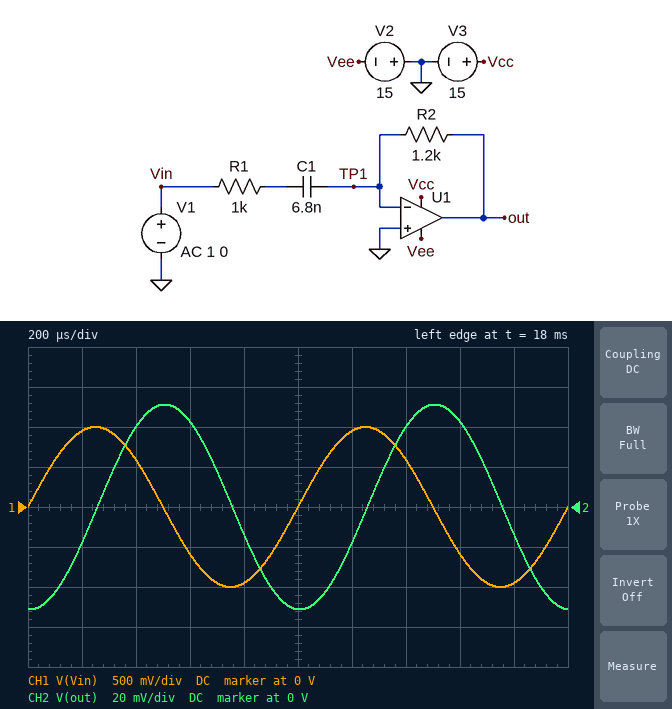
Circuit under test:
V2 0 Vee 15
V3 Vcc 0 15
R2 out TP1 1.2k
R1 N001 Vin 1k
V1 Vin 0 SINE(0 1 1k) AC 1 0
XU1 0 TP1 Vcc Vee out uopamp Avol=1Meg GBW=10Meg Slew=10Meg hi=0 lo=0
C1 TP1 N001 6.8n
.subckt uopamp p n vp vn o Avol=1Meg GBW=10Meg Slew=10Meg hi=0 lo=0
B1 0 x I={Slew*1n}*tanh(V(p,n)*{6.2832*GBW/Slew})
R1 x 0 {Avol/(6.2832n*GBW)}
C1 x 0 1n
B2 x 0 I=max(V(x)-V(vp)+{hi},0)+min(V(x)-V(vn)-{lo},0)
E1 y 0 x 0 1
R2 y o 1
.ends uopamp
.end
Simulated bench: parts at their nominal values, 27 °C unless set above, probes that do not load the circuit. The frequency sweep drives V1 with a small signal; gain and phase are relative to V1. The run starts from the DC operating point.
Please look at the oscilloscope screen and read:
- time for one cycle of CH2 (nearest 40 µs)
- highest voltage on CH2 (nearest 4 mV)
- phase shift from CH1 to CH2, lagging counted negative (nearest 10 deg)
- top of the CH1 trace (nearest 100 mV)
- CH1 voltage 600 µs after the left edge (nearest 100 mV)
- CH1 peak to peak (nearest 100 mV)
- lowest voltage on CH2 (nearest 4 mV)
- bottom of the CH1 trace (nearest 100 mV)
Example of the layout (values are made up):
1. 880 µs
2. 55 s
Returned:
1. 1.00 ms
2. 52 mV
3. -90 deg
4. 1.0 V
5. -600 mV
6. 2.0 V
7. -52 mV
8. -1.0 V
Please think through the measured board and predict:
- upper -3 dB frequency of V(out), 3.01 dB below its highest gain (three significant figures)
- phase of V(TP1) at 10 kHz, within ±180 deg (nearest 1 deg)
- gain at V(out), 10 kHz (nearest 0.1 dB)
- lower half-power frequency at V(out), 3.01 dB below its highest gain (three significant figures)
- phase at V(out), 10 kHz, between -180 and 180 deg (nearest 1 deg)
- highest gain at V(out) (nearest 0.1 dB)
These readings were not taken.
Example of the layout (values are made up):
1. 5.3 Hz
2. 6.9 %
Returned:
1. 4.58 MHz
2. 157 deg
3. -6.5 dB
4. 23.2 kHz
5. -113 deg
6. 1.6 dB
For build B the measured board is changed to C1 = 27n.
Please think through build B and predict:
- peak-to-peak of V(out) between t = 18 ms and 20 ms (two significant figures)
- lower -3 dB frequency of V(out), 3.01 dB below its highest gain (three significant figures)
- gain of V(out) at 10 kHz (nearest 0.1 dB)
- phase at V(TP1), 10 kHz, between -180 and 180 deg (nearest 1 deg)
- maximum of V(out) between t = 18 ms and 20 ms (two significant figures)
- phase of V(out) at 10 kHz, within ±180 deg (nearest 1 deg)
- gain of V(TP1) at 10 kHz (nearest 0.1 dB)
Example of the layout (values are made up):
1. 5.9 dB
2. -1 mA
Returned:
1. 400 mV
2. 5.88 kHz
3. 0.3 dB
4. 120 deg
5. 200 mV
6. -150 deg
7. -59.7 dB
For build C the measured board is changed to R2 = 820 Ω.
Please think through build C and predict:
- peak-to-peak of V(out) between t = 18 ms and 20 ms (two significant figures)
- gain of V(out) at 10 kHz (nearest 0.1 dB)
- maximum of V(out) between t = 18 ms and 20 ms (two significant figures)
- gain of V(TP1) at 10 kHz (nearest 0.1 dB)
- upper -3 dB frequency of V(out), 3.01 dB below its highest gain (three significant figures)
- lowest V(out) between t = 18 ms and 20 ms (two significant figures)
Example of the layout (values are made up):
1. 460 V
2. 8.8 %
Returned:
1. 70 mV
2. -9.8 dB
3. 35 mV
4. -69.8 dB
5. 5.53 MHz
6. -35 mV
